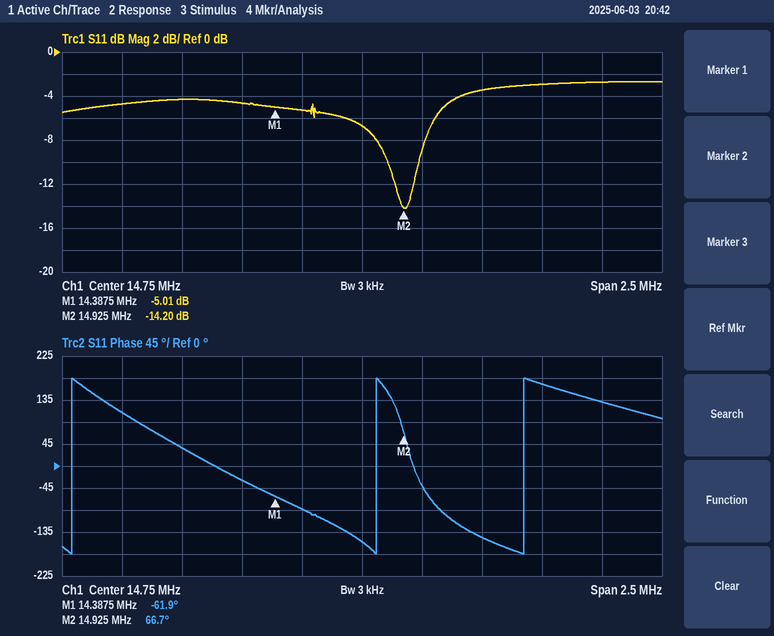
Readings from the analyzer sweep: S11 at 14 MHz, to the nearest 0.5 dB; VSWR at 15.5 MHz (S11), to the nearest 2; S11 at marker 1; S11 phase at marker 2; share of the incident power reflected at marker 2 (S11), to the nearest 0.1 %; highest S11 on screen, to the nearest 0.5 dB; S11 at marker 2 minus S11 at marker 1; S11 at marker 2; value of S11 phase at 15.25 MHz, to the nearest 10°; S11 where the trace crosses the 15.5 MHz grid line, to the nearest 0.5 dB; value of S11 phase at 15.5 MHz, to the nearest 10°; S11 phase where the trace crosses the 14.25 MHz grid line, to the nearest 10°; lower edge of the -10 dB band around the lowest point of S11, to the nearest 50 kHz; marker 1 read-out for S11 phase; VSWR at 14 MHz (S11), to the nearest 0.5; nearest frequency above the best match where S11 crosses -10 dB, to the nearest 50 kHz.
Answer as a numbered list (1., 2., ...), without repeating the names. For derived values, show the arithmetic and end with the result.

1. -4.5 dB
2. |Γ| = 10^(-3/20) = 0.7079; VSWR = (1 + 0.7079)/(1 − 0.7079) ≈ 6
3. -5.01 dB
4. 66.7°
5. 10^(-14.2/10) ≈ 3.8 %
6. -2.5 dB
7. -14.2 − (-5.01) = -9.19 dB
8. -14.20 dB
9. -150°
10. -3.0 dB
11. 170°
12. -30°
13. 14.85 MHz
14. -61.9°
15. |Γ| = 10^(-4.5/20) = 0.5957; VSWR = (1 + 0.5957)/(1 − 0.5957) ≈ 4.0
16. 15.00 MHz
